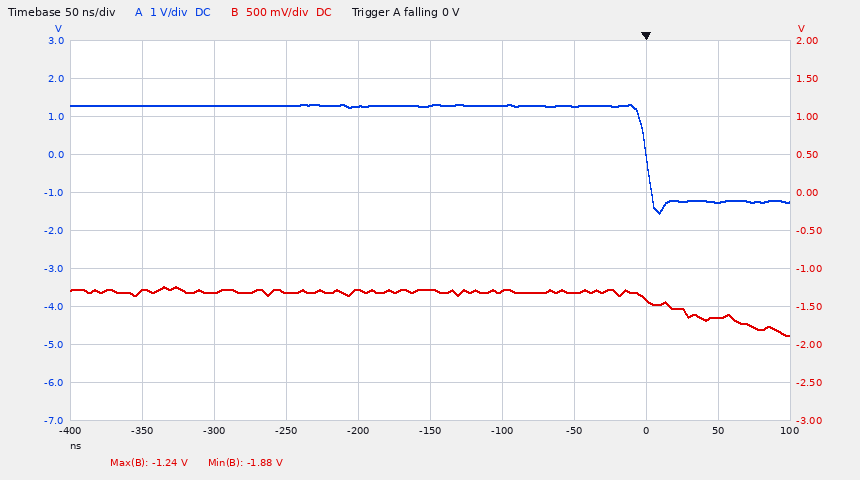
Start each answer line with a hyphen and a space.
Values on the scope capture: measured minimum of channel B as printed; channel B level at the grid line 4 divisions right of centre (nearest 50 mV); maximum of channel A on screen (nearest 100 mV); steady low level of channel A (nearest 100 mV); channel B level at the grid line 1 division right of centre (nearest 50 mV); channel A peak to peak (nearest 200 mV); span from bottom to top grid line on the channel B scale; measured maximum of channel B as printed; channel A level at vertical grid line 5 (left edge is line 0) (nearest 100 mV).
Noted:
- -1.88 V
- -1.65 V
- 1.3 V
- -1.2 V
- -1.30 V
- 2.8 V
- 5 V
- -1.24 V
- 1.3 V
